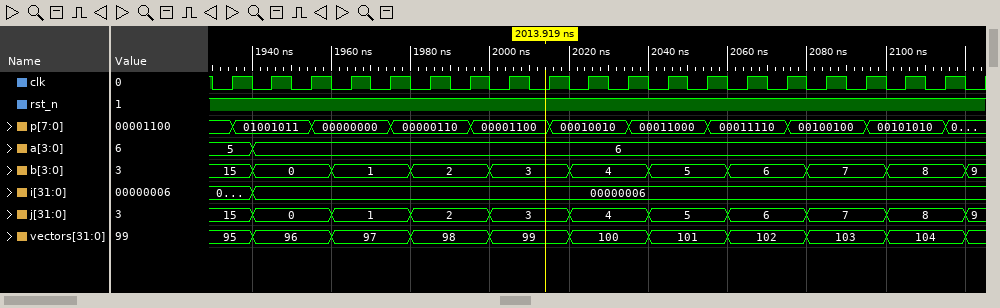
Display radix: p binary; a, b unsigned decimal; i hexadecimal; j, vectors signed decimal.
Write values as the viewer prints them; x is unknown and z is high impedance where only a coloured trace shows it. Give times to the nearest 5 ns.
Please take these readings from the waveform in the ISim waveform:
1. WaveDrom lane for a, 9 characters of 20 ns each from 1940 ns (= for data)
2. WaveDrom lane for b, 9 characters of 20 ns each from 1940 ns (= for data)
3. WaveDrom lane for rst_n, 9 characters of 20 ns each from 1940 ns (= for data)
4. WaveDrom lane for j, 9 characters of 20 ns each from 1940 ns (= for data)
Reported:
{name: 'a', wave: '=........', data: '6'}
{name: 'b', wave: '=========', data: '0 1 2 3 4 5 6 7 8'}
{name: 'rst_n', wave: '1........'}
{name: 'j', wave: '=========', data: '0 1 2 3 4 5 6 7 8'}
